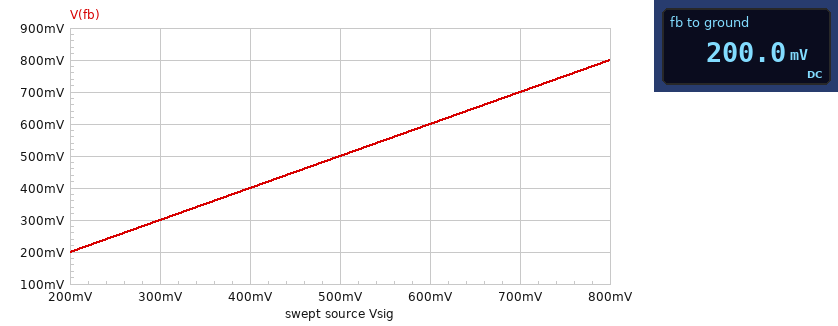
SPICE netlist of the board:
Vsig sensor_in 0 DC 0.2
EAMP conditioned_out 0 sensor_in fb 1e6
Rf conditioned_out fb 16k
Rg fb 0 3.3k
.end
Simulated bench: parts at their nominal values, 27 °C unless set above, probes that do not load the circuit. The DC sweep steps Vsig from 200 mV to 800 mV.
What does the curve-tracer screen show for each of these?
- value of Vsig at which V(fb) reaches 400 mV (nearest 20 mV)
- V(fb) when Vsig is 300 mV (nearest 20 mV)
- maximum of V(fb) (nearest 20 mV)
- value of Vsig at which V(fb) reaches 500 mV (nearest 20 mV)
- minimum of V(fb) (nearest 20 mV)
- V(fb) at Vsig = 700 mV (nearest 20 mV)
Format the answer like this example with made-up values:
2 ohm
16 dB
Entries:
400 mV
300 mV
800 mV
500 mV
200 mV
700 mV
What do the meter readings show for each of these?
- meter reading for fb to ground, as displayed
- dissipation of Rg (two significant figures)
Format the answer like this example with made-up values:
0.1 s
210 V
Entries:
200.0 mV
12 µW
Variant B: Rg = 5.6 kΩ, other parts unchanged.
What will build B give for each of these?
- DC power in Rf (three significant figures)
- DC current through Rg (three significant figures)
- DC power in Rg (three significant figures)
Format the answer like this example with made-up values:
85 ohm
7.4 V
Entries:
20.4 µW
35.7 µA
7.14 µW
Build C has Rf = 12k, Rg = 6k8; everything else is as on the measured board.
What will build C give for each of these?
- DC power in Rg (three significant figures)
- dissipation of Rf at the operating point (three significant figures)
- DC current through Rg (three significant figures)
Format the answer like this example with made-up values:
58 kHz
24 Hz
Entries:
5.88 µW
10.4 µW
29.4 µA
